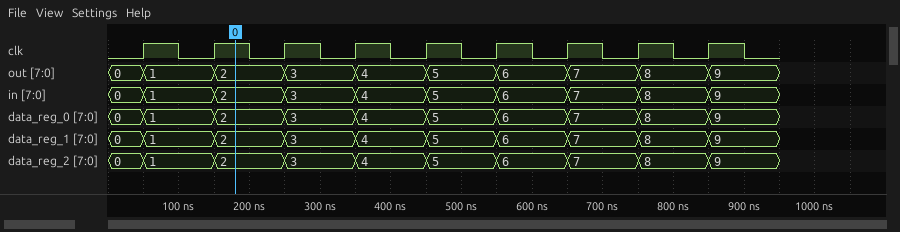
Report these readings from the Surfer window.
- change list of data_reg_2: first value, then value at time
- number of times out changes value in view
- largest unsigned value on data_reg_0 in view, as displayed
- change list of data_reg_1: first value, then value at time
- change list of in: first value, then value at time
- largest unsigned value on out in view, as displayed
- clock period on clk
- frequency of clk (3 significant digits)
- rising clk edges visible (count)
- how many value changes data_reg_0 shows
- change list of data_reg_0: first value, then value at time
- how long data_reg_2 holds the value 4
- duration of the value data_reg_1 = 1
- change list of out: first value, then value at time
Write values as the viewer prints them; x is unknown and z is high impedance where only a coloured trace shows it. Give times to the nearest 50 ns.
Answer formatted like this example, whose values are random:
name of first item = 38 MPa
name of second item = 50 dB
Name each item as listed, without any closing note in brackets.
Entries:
change list of data_reg_2: first value, then value at time = 0, 1 at 50 ns, 2 at 150 ns, 3 at 250 ns, 4 at 350 ns, 5 at 450 ns, 6 at 550 ns, 7 at 650 ns, 8 at 750 ns, 9 at 850 ns
number of times out changes value in view = 9
largest unsigned value on data_reg_0 in view, as displayed = 9
change list of data_reg_1: first value, then value at time = 0, 1 at 50 ns, 2 at 150 ns, 3 at 250 ns, 4 at 350 ns, 5 at 450 ns, 6 at 550 ns, 7 at 650 ns, 8 at 750 ns, 9 at 850 ns
change list of in: first value, then value at time = 0, 1 at 50 ns, 2 at 150 ns, 3 at 250 ns, 4 at 350 ns, 5 at 450 ns, 6 at 550 ns, 7 at 650 ns, 8 at 750 ns, 9 at 850 ns
largest unsigned value on out in view, as displayed = 9
clock period on clk = 100 ns
frequency of clk = 10.0 MHz
rising clk edges visible = 9
how many value changes data_reg_0 shows = 9
change list of data_reg_0: first value, then value at time = 0, 1 at 50 ns, 2 at 150 ns, 3 at 250 ns, 4 at 350 ns, 5 at 450 ns, 6 at 550 ns, 7 at 650 ns, 8 at 750 ns, 9 at 850 ns
how long data_reg_2 holds the value 4 = 100 ns
duration of the value data_reg_1 = 1 = 100 ns
change list of out: first value, then value at time = 0, 1 at 50 ns, 2 at 150 ns, 3 at 250 ns, 4 at 350 ns, 5 at 450 ns, 6 at 550 ns, 7 at 650 ns, 8 at 750 ns, 9 at 850 ns
